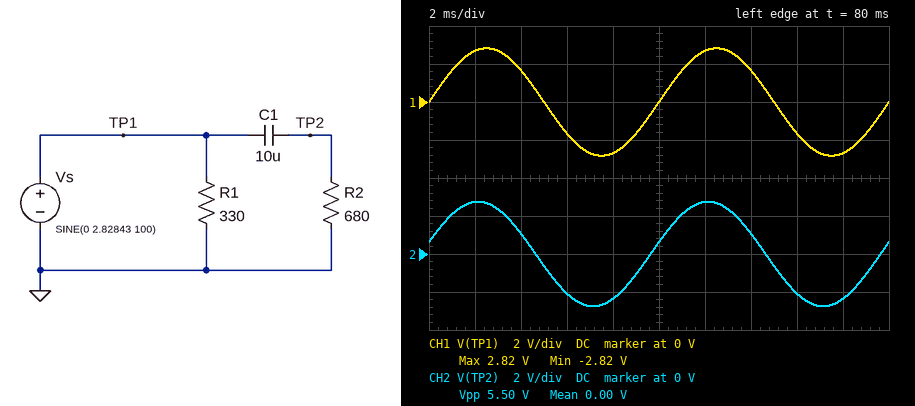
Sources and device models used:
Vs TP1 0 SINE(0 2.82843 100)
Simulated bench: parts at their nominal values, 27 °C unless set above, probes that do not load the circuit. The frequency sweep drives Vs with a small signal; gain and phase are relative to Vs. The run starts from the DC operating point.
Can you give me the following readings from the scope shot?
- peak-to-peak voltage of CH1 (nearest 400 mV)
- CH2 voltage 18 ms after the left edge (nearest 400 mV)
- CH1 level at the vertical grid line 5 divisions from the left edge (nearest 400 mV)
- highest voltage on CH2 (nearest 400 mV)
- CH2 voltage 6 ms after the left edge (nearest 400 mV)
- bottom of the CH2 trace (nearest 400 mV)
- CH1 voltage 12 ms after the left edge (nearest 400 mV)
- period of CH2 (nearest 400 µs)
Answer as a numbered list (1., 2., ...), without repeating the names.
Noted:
1. 5.6 V
2. -2.4 V
3. 0 V
4. 2.8 V
5. -2.0 V
6. -2.8 V
7. 2.8 V
8. 10.0 ms
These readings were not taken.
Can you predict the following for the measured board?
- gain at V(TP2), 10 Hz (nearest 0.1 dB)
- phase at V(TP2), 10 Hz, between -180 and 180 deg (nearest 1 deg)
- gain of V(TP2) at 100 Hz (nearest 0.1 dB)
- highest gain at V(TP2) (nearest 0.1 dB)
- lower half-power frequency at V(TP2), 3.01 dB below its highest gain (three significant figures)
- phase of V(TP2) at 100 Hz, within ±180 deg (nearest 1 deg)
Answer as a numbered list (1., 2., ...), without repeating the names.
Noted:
1. -8.1 dB
2. 67 deg
3. -0.2 dB
4. 0 dB
5. 23.4 Hz
6. 13 deg
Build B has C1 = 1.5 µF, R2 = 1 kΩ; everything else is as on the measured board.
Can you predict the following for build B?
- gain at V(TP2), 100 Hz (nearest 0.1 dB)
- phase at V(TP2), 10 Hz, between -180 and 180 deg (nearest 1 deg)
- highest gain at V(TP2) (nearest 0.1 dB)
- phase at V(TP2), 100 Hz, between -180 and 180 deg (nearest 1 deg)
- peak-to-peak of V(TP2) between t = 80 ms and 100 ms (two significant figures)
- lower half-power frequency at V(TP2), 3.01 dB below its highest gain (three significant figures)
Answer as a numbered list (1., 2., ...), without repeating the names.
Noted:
1. -3.3 dB
2. 85 deg
3. 0 dB
4. 47 deg
5. 3.9 V
6. 106 Hz
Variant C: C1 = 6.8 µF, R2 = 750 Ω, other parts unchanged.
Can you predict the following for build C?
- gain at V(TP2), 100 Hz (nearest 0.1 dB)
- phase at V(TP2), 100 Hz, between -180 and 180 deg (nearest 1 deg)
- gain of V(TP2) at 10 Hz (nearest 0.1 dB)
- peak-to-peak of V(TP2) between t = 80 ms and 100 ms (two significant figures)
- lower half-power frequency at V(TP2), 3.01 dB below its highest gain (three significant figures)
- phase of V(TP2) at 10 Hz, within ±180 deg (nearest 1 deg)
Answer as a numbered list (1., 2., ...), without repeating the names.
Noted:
1. -0.4 dB
2. 17 deg
3. -10.3 dB
4. 5.4 V
5. 31.2 Hz
6. 72 deg
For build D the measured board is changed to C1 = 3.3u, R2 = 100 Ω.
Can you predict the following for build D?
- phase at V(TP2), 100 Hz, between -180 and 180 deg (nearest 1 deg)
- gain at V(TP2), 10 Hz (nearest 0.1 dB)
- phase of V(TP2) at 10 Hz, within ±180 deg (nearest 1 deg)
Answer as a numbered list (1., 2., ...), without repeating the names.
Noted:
1. 78 deg
2. -33.7 dB
3. 89 deg
